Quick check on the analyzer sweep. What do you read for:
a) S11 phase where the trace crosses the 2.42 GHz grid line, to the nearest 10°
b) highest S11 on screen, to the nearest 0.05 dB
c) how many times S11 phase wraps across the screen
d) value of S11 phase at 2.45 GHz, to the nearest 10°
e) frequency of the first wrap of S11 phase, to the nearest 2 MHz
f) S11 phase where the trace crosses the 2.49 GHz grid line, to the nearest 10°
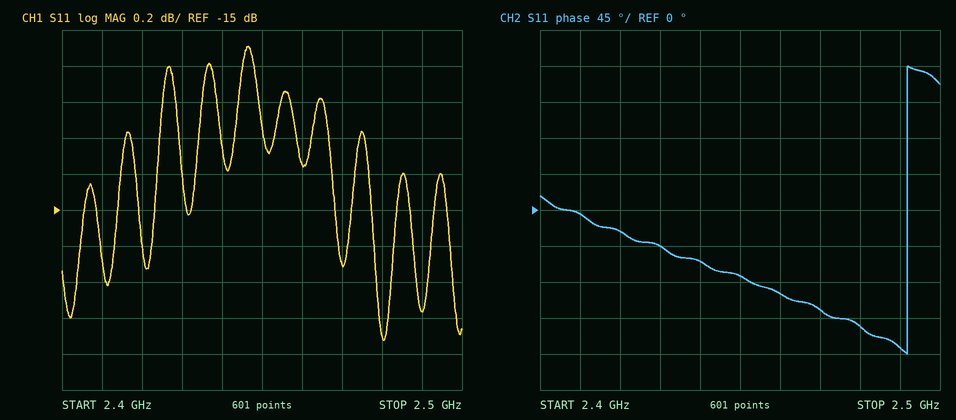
-30°
-14.10 dB
1
-80°
2.492 GHz
-170°
